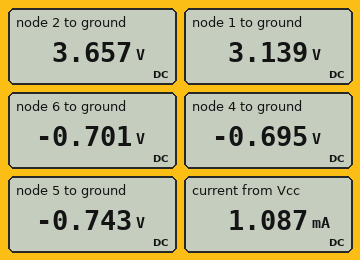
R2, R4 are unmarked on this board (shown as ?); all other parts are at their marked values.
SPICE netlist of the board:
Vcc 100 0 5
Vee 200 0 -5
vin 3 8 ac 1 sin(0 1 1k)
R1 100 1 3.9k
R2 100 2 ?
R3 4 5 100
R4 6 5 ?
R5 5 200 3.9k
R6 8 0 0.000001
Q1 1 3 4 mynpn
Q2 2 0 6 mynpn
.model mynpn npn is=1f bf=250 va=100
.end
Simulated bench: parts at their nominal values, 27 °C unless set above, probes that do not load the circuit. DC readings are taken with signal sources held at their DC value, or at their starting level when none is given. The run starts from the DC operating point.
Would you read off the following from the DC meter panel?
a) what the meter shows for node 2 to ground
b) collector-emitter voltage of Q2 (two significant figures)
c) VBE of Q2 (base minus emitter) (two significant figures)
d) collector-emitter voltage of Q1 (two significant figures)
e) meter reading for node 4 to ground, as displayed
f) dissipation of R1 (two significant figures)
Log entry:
3.657 V
4.4 V
700 mV
3.8 V
-0.695 V
890 µW
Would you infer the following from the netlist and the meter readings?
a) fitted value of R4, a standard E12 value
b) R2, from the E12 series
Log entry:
68 Ω
2.2 kΩ
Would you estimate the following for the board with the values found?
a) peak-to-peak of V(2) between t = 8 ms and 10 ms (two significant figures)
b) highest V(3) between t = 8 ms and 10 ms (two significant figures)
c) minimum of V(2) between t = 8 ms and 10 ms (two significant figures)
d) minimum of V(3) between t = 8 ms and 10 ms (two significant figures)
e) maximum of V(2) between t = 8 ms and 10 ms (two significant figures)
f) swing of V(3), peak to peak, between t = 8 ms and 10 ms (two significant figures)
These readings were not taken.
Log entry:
2.4 V
1.0 V
2.6 V
-1.0 V
5.0 V
2.0 V
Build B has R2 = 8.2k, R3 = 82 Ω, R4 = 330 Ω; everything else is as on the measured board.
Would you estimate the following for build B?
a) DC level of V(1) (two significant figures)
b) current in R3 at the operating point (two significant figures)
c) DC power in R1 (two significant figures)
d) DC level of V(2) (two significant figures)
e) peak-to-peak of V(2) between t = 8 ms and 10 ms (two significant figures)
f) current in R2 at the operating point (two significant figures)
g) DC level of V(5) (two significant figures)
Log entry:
1.9 V
800 µA
2.5 mW
2.7 V
5.7 V
280 µA
-770 mV
